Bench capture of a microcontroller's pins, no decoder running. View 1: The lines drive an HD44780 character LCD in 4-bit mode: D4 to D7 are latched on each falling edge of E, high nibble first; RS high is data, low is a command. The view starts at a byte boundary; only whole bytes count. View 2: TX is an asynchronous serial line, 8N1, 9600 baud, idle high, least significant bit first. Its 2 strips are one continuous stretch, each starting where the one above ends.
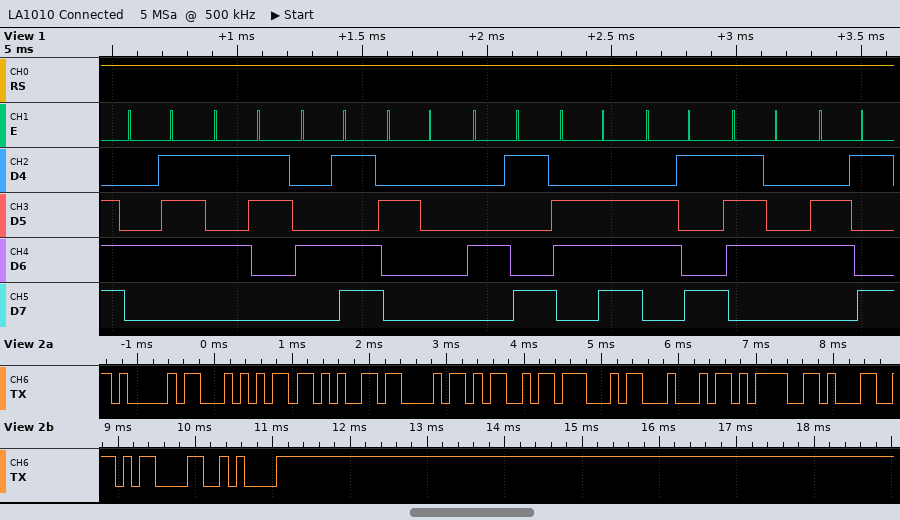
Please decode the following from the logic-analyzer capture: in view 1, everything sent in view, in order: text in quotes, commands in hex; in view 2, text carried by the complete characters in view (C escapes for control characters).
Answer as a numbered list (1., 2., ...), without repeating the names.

1. "GSM Initi"
2. "AT+CMGD=1\r\n"
